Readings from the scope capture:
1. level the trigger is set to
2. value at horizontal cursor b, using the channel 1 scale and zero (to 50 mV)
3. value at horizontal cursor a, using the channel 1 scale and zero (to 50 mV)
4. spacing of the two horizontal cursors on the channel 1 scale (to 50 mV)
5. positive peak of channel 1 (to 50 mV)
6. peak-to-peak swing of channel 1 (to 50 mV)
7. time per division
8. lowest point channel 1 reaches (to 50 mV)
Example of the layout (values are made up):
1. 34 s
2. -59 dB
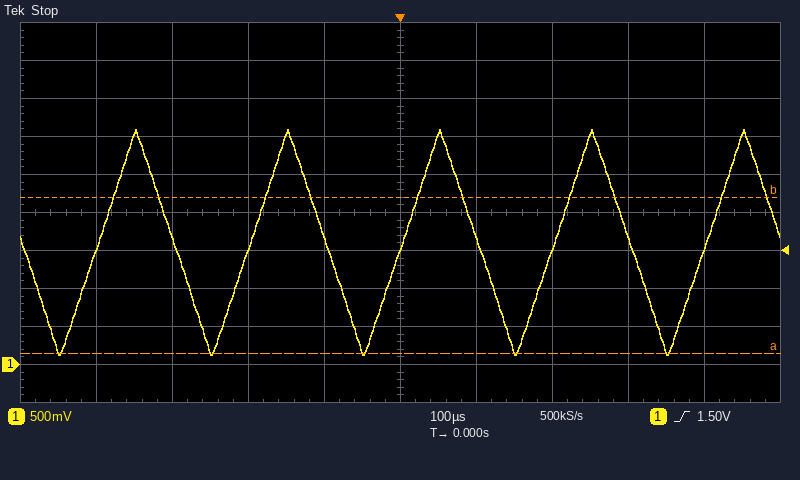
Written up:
1. 1.50 V
2. 2.20 V
3. 150 mV
4. 2.05 V
5. 3.10 V
6. 2.95 V
7. 100 µs
8. 150 mV
